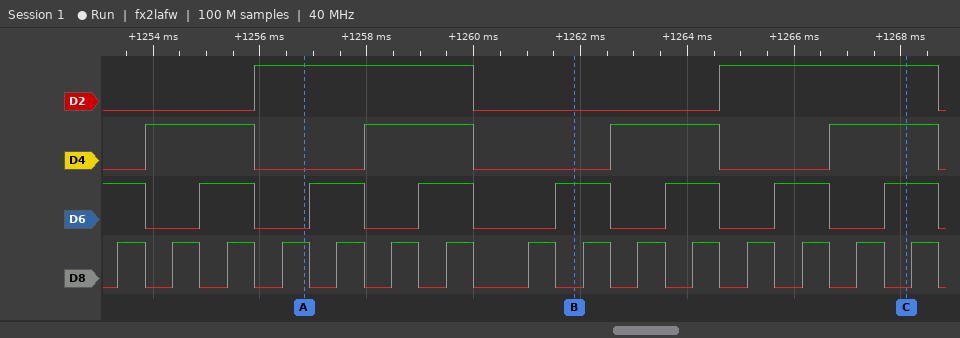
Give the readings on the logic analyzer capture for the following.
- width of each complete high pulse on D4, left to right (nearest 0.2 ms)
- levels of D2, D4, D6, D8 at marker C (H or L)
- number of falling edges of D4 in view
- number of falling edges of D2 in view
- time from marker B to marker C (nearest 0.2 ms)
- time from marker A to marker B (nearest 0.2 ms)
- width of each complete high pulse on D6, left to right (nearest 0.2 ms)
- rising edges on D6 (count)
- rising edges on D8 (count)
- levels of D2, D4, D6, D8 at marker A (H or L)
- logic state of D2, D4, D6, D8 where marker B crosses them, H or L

2 ms, 2 ms, 2 ms, 2 ms
D2=H, D4=H, D6=H, D8=L
4
2
6.2 ms
5 ms
1 ms, 1 ms, 1 ms, 1 ms, 1 ms, 1 ms, 1 ms
7
15
D2=H, D4=L, D6=L, D8=H
D2=L, D4=L, D6=H, D8=L
